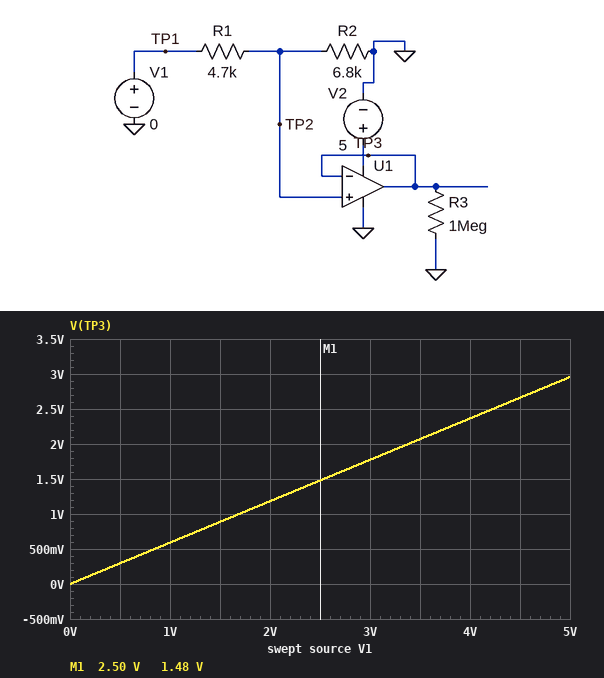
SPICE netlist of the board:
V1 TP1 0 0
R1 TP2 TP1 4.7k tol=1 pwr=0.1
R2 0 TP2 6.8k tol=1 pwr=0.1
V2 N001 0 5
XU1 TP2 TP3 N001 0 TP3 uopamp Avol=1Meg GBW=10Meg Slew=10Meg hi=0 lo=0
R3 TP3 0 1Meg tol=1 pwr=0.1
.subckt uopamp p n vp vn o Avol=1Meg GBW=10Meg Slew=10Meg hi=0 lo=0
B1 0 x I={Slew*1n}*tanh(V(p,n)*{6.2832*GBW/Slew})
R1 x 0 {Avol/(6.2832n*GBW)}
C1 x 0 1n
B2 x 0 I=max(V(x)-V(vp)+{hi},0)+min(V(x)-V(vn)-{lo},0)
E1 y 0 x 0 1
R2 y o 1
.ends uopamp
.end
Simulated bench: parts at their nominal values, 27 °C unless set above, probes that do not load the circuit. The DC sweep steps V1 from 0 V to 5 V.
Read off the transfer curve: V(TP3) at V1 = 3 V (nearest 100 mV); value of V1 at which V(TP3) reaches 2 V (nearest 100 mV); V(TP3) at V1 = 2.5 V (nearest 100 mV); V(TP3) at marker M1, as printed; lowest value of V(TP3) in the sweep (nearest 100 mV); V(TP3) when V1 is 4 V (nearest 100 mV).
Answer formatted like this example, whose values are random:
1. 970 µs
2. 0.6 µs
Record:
1. 1.8 V
2. 3.4 V
3. 1.5 V
4. 1.48 V
5. 0 V
6. 2.4 V
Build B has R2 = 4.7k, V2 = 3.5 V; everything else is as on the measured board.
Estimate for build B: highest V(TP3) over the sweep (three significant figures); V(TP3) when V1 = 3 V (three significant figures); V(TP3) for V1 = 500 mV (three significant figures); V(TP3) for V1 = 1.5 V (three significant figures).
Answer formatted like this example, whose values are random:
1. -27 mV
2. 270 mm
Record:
1. 2.50 V
2. 1.50 V
3. 250 mV
4. 750 mV
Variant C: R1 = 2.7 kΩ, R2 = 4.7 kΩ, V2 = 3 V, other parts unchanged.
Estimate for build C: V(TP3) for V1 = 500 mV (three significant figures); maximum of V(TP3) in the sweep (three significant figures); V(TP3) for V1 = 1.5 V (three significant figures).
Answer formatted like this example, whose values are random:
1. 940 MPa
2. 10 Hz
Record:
1. 318 mV
2. 3.01 V
3. 953 mV
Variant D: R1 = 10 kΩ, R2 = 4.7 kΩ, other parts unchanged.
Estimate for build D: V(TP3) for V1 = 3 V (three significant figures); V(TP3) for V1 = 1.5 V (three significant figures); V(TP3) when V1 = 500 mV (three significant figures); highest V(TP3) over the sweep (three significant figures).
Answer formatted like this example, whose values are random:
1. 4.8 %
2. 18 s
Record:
1. 959 mV
2. 480 mV
3. 160 mV
4. 1.60 V
